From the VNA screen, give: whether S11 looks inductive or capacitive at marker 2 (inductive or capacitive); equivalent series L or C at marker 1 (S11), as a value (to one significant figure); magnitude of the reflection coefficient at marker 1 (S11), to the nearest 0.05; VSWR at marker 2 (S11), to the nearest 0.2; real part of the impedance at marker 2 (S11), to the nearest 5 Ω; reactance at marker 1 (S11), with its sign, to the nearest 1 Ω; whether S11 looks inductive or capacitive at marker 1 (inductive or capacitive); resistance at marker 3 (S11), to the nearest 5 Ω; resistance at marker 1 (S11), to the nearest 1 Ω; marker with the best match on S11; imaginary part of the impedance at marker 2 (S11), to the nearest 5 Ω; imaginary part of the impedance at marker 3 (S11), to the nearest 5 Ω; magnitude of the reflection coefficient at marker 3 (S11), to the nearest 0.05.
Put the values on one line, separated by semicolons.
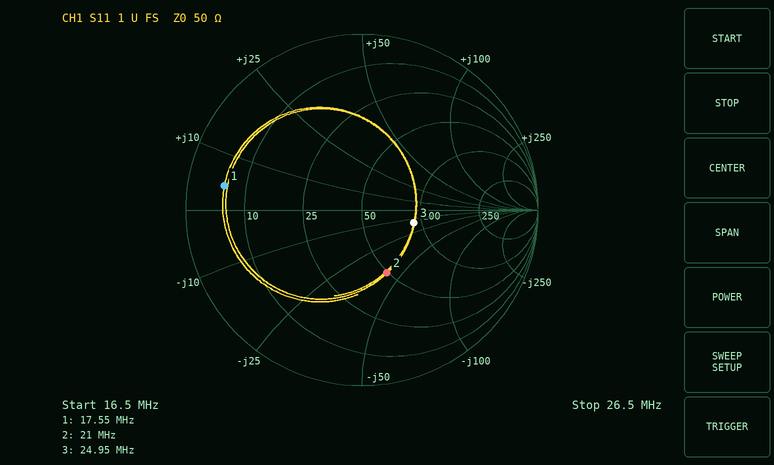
capacitive; 40 nH; 0.80; 2.2; 50 Ω; +4 Ω; inductive; 90 Ω; 6 Ω; marker 3; -40 Ω; -15 Ω; 0.30
